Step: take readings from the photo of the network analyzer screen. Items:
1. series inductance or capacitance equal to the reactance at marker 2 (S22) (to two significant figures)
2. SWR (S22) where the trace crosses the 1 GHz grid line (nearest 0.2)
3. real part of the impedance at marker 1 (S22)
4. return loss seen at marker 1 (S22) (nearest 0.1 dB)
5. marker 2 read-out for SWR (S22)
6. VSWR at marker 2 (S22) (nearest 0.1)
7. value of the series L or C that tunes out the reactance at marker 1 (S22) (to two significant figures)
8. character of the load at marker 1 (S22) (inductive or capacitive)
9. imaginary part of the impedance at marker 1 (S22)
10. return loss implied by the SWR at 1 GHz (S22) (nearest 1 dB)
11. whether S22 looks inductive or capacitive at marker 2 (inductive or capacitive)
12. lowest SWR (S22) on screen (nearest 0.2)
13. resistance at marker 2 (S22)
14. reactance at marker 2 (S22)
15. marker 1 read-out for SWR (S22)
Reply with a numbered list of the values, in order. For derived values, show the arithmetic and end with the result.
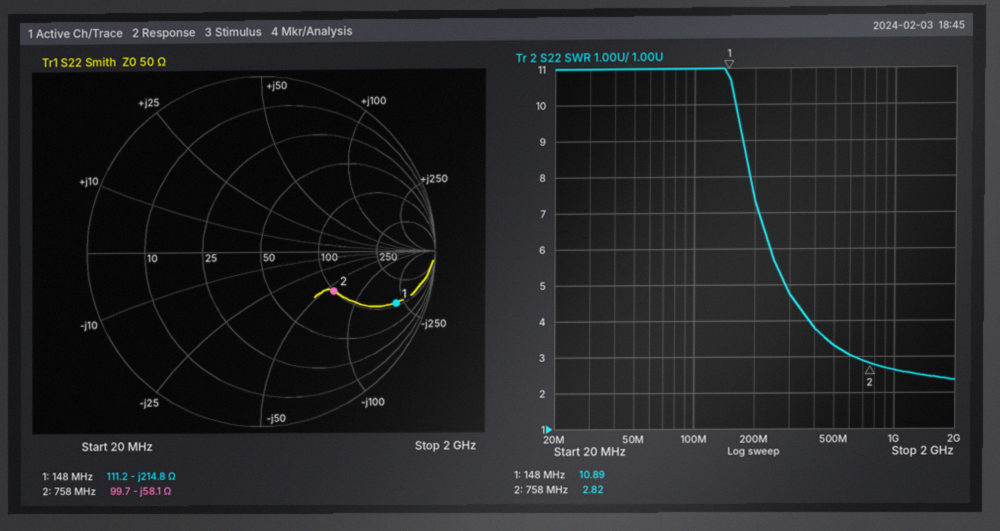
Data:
1. C = 1/(2π × 758 MHz × 58.1 Ω) ≈ 3.6 pF
2. 2.6
3. 111.2 Ω
4. 1.6 dB
5. 2.82
6. 2.8
7. L = 214.8 Ω/(2π × 148 MHz) ≈ 231 nH, so 230 nH to two significant figures
8. capacitive
9. -214.8 Ω
10. −20 log10((2.6 − 1)/(2.6 + 1)) ≈ 7 dB
11. capacitive
12. 2.4
13. 99.7 Ω
14. -58.1 Ω
15. 10.89
